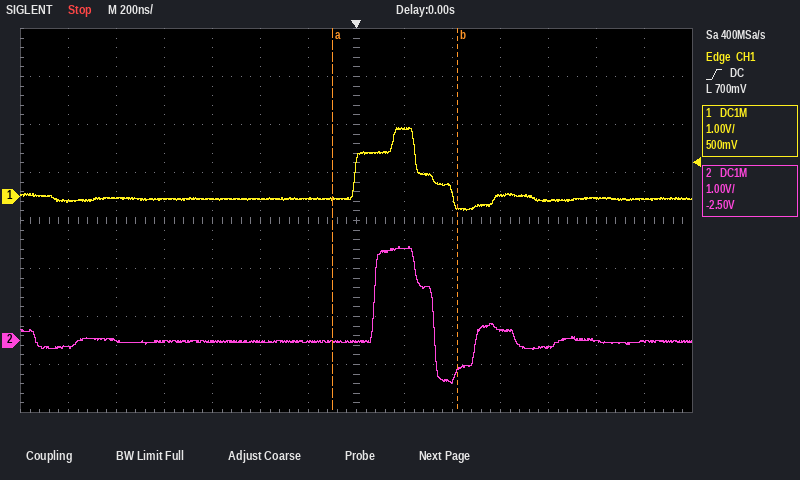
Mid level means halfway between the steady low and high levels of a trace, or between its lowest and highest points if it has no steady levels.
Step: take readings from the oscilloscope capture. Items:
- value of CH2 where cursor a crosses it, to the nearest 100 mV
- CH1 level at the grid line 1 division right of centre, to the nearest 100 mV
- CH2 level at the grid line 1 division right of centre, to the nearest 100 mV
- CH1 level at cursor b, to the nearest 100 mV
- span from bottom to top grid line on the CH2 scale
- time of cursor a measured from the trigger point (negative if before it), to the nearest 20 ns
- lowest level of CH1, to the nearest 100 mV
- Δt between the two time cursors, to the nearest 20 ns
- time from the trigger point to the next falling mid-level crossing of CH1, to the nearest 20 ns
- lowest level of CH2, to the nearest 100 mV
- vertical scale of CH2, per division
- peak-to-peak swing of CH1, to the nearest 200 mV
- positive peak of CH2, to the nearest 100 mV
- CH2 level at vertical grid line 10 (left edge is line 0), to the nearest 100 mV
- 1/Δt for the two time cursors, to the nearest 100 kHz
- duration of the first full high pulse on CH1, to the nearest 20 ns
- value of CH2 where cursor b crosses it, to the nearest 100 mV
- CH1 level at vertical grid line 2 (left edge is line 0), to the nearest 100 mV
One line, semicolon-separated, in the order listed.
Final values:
0.0 V; 1.4 V; 1.9 V; -200 mV; 8 V; -100 ns; -300 mV; 520 ns; 260 ns; -900 mV; 1 V; 1.8 V; 2.0 V; 200 mV; 1.9 MHz; 260 ns; -700 mV; 0.0 V
